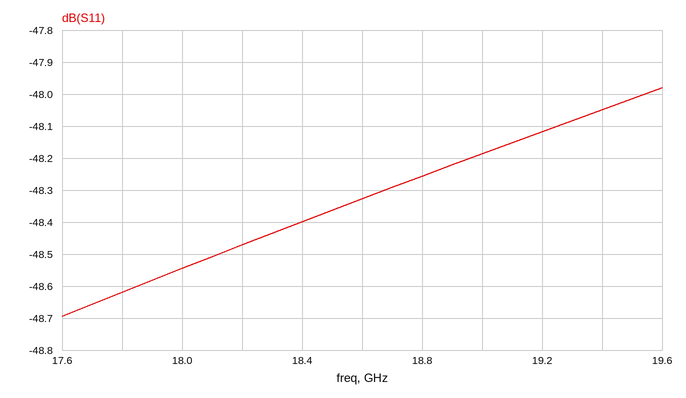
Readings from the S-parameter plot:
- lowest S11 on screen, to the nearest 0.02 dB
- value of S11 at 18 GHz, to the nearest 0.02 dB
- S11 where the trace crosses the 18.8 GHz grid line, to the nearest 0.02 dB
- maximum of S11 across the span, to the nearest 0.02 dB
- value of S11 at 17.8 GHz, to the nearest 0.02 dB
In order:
-48.70 dB
-48.54 dB
-48.26 dB
-47.98 dB
-48.62 dB
